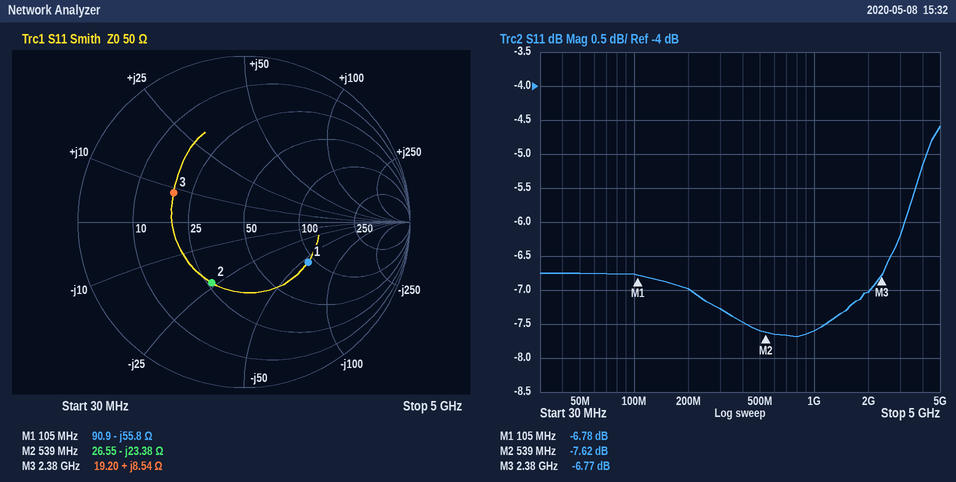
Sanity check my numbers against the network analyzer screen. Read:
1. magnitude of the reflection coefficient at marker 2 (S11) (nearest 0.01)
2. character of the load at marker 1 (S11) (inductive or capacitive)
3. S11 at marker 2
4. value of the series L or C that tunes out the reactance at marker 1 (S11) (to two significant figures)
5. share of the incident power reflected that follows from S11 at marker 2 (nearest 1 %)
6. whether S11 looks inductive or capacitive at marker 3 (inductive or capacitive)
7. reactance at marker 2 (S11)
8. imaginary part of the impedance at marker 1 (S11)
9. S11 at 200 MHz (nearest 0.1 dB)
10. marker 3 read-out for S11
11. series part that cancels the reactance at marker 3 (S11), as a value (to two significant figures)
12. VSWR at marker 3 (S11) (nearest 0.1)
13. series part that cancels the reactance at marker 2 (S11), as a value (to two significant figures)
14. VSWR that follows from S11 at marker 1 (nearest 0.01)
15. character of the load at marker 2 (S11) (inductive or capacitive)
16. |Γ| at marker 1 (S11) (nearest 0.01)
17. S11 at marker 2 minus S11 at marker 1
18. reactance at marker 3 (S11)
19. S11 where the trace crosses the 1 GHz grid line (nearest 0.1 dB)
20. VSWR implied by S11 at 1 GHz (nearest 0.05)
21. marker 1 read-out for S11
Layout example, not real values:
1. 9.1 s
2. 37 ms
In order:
1. 0.41
2. capacitive
3. -7.62 dB
4. 85 nH
5. 17 %
6. inductive
7. -23.38 Ω
8. -55.8 Ω
9. -7.0 dB
10. -6.77 dB
11. 7.8 pF
12. 2.7
13. 6.9 nH
14. 2.69
15. capacitive
16. 0.46
17. -0.84 dB
18. +8.54 Ω
19. -7.6 dB
20. 2.45
21. -6.78 dB
